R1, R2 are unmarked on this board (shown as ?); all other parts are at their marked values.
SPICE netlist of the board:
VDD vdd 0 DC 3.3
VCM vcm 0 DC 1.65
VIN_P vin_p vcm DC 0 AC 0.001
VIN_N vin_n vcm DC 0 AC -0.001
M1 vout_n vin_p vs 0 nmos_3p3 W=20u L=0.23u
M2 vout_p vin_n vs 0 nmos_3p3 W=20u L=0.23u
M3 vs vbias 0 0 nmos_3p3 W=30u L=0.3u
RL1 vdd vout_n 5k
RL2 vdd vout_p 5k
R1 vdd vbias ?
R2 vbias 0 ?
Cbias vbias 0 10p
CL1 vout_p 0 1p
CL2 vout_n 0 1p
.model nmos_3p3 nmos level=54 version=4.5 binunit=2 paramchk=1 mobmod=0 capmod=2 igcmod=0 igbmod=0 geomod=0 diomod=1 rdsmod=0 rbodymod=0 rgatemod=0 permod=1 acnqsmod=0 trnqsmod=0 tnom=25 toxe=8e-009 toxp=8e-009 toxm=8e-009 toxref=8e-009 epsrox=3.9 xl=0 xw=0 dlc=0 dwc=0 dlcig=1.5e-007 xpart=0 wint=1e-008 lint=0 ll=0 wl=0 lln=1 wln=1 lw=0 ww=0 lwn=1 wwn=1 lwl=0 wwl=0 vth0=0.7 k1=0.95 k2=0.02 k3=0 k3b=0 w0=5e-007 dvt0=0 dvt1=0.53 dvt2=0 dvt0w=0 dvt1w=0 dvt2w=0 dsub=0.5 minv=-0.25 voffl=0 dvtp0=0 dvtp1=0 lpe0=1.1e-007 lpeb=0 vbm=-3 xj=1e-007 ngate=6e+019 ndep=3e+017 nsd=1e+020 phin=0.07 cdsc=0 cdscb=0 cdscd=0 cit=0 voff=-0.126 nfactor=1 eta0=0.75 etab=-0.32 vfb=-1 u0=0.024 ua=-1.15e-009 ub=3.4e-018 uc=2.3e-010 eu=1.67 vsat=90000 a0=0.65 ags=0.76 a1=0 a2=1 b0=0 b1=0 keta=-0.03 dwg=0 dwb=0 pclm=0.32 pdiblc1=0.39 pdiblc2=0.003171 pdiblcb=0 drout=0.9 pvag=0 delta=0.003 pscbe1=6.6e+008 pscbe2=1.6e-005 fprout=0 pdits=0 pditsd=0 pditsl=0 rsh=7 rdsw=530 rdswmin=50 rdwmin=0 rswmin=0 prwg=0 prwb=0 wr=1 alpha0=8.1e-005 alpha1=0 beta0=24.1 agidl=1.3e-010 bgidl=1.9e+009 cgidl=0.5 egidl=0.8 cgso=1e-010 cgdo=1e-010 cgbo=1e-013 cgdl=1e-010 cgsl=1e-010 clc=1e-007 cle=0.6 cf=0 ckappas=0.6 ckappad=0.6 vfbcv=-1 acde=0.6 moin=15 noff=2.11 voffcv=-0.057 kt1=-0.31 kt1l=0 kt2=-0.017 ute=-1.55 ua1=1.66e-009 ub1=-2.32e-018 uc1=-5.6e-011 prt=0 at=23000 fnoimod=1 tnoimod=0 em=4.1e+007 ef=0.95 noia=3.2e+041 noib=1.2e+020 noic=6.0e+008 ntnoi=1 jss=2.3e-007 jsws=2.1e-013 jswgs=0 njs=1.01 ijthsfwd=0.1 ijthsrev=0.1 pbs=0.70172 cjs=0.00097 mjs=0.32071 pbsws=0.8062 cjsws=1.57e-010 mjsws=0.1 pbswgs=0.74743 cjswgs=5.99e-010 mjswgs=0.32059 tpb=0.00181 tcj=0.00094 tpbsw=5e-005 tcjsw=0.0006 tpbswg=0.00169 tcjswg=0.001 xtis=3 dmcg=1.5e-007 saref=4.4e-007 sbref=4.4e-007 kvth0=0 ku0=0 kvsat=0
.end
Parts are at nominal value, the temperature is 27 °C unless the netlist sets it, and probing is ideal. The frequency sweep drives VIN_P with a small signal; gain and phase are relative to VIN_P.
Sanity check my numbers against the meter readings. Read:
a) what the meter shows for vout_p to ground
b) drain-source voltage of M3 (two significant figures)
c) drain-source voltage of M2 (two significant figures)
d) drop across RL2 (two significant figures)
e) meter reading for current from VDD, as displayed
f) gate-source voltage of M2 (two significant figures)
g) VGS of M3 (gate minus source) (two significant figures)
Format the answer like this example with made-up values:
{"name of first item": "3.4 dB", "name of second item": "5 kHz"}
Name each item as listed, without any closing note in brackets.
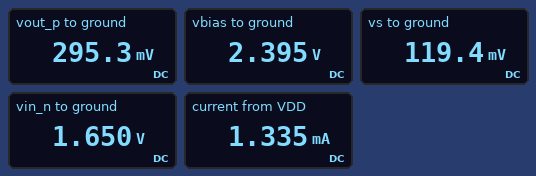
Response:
{"what the meter shows for vout_p to ground": "295.3 mV", "drain-source voltage of M3": "120 mV", "drain-source voltage of M2": "180 mV", "drop across RL2": "3.0 V", "meter reading for current from VDD, as displayed": "1.335 mA", "gate-source voltage of M2": "1.5 V", "VGS of M3 (gate minus source)": "2.4 V"}
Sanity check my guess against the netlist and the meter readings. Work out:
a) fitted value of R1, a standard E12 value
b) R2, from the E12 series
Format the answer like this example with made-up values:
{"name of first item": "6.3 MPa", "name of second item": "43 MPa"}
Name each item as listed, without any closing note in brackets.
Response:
{"fitted value of R1, a standard E12 value": "6.8 kΩ", "R2, from the E12 series": "18 kΩ"}
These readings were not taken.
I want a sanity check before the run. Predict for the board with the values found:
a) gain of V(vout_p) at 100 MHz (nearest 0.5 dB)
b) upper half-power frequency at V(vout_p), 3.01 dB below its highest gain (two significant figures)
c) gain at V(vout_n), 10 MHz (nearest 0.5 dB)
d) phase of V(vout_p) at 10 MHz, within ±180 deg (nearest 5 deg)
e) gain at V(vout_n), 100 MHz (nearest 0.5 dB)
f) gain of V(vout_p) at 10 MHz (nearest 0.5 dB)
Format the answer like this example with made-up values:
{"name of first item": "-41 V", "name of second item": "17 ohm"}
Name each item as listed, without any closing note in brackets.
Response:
{"gain of V(vout_p) at 100 MHz": "-28.5 dB", "upper half-power frequency at V(vout_p), 3.01 dB below its highest gain": "790 MHz", "gain at V(vout_n), 10 MHz": "-8.5 dB", "phase of V(vout_p) at 10 MHz, within ±180 deg": "15 deg", "gain at V(vout_n), 100 MHz": "-9.0 dB", "gain of V(vout_p) at 10 MHz": "-38.0 dB"}
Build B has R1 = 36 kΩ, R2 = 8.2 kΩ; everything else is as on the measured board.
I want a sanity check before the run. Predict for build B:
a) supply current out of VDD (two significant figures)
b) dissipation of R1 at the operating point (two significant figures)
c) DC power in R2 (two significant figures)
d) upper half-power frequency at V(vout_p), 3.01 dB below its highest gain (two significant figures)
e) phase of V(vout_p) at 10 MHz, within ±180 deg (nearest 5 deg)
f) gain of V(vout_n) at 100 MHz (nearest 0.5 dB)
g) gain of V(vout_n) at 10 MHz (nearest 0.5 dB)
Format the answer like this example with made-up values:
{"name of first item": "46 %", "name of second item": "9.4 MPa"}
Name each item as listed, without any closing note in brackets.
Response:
{"supply current out of VDD": "75 µA", "dissipation of R1 at the operating point": "200 µW", "DC power in R2": "46 µW", "upper half-power frequency at V(vout_p), 3.01 dB below its highest gain": "11 MHz", "phase of V(vout_p) at 10 MHz, within ±180 deg": "-50 deg", "gain of V(vout_n) at 100 MHz": "-48.5 dB", "gain of V(vout_n) at 10 MHz": "-43.5 dB"}
